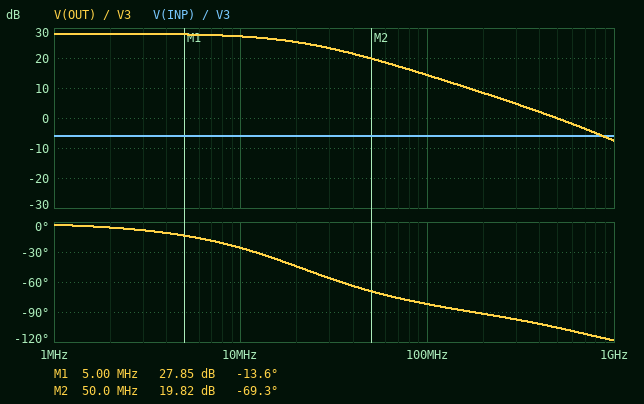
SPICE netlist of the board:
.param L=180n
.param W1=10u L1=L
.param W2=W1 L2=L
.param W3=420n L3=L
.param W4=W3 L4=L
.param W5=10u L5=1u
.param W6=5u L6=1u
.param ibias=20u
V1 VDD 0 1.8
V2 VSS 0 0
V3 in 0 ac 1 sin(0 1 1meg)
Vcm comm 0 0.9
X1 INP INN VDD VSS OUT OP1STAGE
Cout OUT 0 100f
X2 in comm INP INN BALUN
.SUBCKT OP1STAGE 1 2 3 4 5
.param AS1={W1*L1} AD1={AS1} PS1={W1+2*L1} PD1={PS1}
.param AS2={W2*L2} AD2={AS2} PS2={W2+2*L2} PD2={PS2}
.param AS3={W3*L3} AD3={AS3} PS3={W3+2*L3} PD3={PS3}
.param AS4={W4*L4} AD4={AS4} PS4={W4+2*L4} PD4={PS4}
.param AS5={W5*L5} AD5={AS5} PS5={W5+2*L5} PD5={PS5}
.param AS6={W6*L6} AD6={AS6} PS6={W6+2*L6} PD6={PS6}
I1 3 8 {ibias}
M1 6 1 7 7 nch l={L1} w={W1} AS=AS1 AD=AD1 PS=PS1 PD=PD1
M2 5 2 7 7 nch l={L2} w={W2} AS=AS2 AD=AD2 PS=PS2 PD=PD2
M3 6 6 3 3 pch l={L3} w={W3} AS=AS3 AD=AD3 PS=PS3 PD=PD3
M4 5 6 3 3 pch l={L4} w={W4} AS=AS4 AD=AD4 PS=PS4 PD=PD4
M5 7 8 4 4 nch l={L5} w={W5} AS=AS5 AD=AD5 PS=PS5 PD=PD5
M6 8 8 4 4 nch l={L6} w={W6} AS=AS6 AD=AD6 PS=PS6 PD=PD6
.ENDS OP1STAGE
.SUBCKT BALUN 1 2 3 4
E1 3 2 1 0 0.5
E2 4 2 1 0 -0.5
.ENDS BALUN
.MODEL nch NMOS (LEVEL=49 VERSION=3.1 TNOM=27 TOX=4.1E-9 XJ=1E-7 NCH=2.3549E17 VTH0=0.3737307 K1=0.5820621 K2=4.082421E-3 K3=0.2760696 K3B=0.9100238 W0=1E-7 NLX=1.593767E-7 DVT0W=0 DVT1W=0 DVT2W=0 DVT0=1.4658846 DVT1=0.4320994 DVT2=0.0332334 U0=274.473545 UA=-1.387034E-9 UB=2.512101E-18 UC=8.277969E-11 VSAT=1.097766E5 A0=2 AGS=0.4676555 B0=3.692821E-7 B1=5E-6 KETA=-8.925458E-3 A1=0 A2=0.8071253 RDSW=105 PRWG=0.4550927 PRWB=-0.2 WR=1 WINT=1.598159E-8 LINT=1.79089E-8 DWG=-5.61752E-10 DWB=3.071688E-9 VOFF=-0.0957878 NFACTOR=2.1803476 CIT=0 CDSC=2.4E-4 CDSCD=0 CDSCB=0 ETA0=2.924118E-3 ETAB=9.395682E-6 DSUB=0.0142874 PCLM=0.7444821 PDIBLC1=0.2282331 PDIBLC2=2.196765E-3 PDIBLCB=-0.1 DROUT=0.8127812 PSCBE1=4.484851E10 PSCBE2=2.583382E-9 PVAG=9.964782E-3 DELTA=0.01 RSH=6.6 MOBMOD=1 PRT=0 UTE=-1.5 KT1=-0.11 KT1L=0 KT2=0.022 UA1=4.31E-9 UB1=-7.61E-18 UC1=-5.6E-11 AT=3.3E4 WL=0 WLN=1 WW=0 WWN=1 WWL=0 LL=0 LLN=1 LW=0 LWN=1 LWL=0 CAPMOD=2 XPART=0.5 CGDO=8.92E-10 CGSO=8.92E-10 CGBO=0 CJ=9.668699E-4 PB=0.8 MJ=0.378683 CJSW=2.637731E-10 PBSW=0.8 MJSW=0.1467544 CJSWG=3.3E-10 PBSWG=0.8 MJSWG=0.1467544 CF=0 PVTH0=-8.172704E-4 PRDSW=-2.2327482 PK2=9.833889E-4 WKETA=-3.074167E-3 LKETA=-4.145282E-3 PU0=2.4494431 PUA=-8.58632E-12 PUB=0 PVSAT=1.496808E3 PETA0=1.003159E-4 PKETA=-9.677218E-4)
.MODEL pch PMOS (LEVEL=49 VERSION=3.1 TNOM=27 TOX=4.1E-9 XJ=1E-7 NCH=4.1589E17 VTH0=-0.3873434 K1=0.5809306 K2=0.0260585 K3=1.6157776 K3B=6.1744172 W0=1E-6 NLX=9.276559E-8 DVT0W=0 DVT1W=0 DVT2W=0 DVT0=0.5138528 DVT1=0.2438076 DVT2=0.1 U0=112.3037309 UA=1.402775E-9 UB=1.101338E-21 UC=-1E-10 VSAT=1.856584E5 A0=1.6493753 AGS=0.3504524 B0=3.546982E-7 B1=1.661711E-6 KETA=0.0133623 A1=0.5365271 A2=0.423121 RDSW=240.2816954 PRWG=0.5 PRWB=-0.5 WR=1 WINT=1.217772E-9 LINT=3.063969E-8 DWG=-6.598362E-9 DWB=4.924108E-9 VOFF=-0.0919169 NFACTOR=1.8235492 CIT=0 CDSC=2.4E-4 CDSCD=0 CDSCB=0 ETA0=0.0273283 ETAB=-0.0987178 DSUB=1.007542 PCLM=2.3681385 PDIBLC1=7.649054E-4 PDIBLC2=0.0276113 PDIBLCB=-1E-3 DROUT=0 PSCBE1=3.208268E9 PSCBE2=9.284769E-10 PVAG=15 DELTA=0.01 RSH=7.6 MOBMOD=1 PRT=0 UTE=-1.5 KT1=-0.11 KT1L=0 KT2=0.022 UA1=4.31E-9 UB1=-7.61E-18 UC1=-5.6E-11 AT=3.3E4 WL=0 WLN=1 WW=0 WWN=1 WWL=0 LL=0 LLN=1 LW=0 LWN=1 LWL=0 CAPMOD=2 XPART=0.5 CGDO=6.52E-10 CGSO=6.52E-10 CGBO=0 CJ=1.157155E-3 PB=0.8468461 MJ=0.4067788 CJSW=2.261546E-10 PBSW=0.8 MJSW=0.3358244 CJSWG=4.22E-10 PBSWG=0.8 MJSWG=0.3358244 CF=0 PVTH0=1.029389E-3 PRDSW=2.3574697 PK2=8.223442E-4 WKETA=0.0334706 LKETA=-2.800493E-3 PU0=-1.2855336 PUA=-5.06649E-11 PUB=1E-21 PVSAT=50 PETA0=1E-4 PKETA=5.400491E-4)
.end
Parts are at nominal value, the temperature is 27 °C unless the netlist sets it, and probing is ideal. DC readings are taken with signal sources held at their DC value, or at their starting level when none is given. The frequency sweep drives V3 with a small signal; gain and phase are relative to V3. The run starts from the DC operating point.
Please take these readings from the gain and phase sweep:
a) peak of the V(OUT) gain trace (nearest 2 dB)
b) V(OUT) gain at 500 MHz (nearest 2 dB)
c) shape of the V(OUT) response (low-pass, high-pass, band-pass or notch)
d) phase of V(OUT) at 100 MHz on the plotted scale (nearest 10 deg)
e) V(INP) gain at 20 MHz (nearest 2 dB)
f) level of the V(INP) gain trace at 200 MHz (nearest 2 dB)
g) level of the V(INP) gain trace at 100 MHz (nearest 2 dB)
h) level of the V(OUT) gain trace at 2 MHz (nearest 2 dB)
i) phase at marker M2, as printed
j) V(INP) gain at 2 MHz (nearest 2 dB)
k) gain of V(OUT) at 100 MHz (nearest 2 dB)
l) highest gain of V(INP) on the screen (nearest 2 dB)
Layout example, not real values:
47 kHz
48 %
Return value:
28 dB
0 dB
low-pass
-80 deg
-6 dB
-6 dB
-6 dB
28 dB
-69.3 deg
-6 dB
14 dB
-6 dB
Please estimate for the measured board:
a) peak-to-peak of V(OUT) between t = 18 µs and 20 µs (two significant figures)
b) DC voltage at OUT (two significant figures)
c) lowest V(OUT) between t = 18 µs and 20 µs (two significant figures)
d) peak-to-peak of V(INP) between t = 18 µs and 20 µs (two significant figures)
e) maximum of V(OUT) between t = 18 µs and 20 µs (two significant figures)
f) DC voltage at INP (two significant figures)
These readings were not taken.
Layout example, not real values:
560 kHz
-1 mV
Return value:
1.8 V
900 mV
15 mV
1.0 V
1.8 V
900 mV
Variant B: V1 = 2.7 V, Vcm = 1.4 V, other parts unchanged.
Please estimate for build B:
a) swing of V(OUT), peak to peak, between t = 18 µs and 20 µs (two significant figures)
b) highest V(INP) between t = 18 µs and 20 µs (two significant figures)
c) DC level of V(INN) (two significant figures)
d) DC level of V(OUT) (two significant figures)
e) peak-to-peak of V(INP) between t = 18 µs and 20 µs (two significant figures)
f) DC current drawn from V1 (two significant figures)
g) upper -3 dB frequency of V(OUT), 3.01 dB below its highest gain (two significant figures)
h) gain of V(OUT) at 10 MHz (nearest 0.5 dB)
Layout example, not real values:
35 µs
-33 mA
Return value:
2.3 V
1.9 V
1.4 V
1.8 V
1.0 V
61 µA
20 MHz
28.0 dB
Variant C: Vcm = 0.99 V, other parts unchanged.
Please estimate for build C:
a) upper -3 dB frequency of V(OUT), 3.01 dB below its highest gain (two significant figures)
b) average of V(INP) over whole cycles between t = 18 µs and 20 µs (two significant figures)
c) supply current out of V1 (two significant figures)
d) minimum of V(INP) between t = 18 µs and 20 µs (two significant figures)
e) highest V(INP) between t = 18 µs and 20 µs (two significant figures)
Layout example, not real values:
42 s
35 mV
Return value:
22 MHz
990 mV
60 µA
490 mV
1.5 V
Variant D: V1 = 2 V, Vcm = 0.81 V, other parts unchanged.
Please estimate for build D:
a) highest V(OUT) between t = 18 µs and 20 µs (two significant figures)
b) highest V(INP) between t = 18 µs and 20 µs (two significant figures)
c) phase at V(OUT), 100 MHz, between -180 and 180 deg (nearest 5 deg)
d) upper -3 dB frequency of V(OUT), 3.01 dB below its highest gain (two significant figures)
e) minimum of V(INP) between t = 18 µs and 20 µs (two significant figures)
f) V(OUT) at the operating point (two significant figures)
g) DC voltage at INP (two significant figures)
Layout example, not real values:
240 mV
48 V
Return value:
2.0 V
1.3 V
-85 deg
19 MHz
310 mV
1.1 V
810 mV
